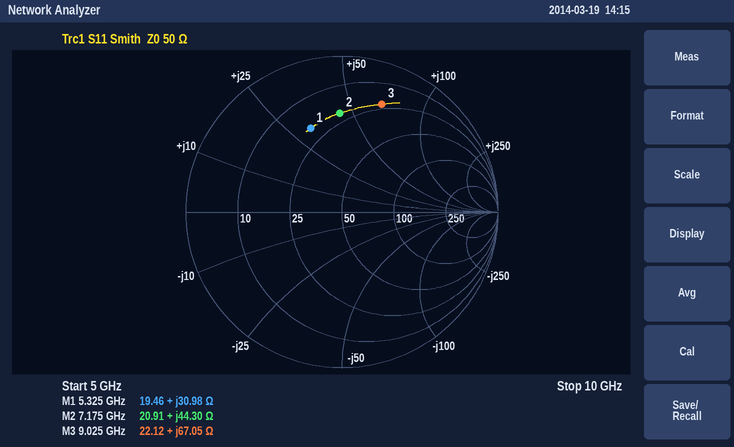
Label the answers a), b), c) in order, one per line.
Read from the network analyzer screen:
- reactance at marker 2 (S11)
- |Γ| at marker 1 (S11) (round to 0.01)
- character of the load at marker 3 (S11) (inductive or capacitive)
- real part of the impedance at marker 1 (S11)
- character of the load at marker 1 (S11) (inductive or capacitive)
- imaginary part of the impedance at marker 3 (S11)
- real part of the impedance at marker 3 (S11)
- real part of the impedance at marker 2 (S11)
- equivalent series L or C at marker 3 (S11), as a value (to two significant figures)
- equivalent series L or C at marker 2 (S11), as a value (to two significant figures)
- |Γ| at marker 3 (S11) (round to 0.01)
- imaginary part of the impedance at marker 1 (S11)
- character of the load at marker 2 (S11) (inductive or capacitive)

a) +44.30 Ω
b) 0.57
c) inductive
d) 19.46 Ω
e) inductive
f) +67.05 Ω
g) 22.12 Ω
h) 20.91 Ω
i) 1.2 nH
j) 980 pH
k) 0.74
l) +30.98 Ω
m) inductive
